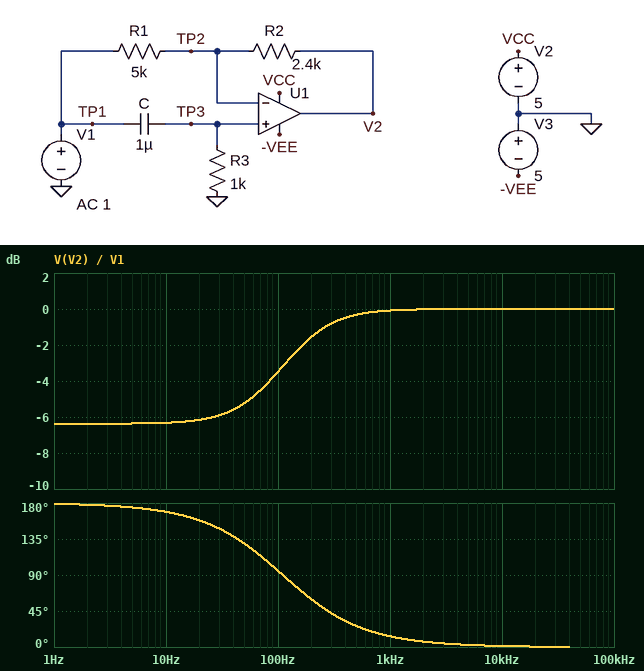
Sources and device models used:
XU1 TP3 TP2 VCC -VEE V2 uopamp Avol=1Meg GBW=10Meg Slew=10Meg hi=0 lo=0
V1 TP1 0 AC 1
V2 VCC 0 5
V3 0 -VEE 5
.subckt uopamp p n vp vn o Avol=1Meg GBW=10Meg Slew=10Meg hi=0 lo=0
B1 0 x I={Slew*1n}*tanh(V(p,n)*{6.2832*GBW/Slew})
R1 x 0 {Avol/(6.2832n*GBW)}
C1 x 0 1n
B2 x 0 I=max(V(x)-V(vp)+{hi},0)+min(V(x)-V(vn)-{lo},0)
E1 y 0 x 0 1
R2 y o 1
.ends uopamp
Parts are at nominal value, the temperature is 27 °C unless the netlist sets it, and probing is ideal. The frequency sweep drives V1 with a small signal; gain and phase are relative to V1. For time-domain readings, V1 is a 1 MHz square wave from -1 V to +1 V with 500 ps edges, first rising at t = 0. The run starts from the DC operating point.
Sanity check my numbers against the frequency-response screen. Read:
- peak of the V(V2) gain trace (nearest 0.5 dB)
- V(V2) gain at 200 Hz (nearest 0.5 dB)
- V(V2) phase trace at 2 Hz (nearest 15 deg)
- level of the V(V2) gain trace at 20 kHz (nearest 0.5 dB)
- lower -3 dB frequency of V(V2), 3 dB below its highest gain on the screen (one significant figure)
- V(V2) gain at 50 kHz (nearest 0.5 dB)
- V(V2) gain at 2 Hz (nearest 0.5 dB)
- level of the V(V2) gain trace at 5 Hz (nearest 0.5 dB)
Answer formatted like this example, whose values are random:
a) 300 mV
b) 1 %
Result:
a) 0 dB
b) -1.5 dB
c) 180 deg
d) 0 dB
e) 100 Hz
f) 0 dB
g) -6.5 dB
h) -6.5 dB
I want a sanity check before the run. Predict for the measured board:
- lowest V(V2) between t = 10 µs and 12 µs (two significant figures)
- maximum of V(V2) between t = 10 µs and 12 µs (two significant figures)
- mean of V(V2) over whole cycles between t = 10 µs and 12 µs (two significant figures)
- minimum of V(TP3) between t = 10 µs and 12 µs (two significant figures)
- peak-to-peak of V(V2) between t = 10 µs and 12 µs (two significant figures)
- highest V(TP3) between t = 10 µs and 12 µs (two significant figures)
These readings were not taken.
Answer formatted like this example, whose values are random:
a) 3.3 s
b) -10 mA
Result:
a) 460 mV
b) 2.5 V
c) 1.5 V
d) -12 mV
e) 2.0 V
f) 2.0 V
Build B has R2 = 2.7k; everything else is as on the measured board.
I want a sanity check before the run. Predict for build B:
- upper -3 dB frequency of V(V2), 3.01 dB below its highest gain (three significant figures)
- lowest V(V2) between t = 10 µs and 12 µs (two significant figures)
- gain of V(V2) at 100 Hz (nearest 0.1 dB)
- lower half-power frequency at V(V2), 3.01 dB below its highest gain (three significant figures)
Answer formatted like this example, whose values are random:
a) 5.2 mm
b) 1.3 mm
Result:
a) 6.49 MHz
b) 520 mV
c) -3.1 dB
d) 103 Hz
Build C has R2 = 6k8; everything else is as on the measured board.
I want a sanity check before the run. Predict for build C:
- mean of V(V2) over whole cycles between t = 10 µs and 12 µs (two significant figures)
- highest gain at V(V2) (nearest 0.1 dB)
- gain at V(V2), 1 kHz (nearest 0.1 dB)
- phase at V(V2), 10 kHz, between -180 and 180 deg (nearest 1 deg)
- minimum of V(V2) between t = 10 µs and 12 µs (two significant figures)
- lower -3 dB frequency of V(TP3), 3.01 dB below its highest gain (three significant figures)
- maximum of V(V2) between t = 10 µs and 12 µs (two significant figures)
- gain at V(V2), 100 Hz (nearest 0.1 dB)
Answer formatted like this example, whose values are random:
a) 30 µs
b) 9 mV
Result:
a) 2.3 V
b) 2.7 dB
c) 0.1 dB
d) 2 deg
e) 1.3 V
f) 159 Hz
g) 3.3 V
h) 2.1 dB
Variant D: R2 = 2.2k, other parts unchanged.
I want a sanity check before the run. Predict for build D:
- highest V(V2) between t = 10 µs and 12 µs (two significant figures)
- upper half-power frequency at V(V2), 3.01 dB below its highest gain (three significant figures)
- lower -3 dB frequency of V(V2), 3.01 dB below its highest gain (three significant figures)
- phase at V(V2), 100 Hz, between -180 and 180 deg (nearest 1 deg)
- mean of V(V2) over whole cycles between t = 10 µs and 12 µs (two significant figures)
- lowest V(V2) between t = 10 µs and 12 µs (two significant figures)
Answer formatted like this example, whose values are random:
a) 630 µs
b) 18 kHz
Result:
a) 2.4 V
b) 6.94 MHz
c) 125 Hz
d) 93 deg
e) 1.4 V
f) 420 mV
